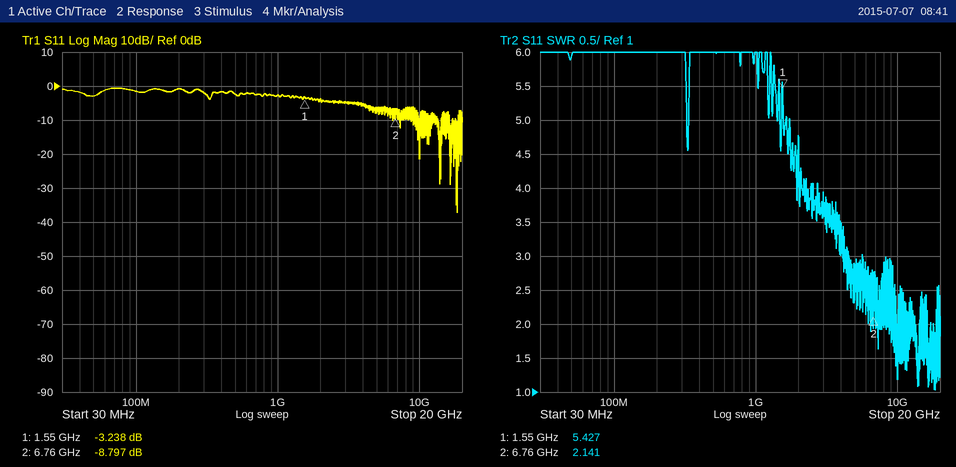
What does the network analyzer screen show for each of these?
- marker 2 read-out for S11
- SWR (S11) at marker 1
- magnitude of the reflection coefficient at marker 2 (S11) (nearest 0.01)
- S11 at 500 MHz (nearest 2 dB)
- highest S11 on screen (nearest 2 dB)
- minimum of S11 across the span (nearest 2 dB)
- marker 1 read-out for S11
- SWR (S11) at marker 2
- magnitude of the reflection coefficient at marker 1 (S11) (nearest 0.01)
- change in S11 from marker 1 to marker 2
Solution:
-8.797 dB
5.427
0.36
-2 dB
0 dB
-38 dB
-3.238 dB
2.141
0.69
-5.559 dB
